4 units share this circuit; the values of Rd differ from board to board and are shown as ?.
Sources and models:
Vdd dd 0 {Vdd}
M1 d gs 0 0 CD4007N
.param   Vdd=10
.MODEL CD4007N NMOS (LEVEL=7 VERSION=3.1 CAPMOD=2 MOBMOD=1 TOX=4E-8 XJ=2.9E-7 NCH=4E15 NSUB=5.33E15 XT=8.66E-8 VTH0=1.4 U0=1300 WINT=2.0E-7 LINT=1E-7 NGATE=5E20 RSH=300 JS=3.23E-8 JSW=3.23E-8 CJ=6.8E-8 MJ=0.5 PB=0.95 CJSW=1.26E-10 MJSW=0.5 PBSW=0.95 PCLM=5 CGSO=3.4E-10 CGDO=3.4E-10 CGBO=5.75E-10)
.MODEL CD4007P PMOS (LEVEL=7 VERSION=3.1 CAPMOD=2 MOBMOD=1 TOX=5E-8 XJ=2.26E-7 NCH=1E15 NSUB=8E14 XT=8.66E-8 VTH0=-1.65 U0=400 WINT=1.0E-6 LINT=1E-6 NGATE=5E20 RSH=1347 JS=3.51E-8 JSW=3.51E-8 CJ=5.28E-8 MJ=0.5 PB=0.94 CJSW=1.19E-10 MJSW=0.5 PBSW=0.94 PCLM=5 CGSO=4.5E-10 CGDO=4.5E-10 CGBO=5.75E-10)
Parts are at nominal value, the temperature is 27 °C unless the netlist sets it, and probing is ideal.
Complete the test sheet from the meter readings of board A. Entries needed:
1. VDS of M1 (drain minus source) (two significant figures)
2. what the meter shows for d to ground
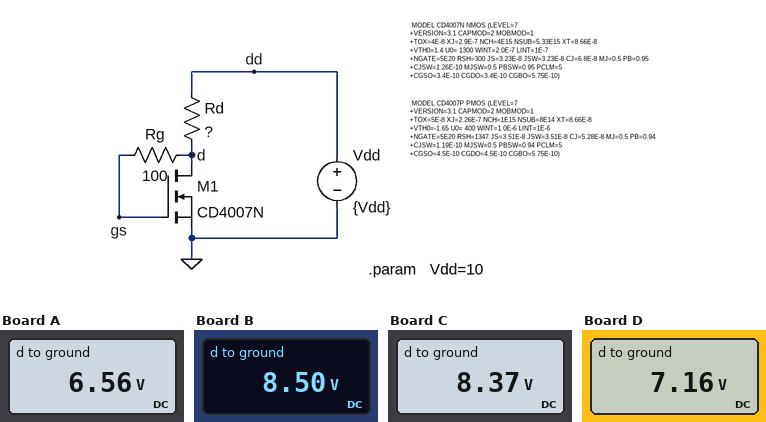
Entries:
6.6 V
6.56 V
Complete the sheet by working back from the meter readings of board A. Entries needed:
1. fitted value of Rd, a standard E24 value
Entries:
6.8 kΩ
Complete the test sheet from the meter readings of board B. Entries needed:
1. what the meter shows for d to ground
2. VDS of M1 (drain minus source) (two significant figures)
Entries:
8.50 V
8.5 V
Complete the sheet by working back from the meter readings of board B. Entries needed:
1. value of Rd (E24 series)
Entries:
1.8 kΩ
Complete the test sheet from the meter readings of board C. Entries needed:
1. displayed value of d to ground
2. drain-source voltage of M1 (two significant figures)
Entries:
8.37 V
8.4 V
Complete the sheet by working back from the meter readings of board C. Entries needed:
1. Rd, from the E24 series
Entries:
2 kΩ
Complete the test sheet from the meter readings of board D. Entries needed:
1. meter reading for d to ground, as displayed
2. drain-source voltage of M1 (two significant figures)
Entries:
7.16 V
7.2 V
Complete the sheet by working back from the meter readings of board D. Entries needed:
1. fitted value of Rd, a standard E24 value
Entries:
4.7 kΩ
